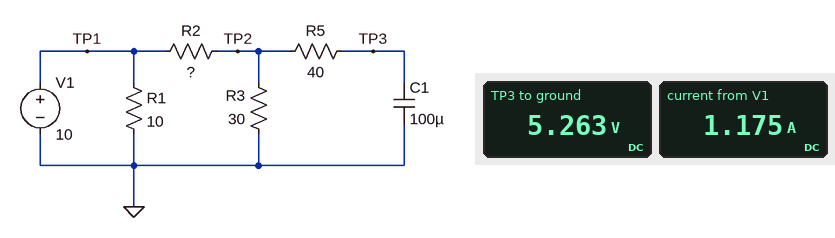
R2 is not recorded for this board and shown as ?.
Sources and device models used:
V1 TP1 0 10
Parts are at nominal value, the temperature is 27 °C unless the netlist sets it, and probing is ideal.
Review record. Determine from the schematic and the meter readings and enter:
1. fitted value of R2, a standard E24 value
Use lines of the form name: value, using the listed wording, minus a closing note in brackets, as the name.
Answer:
fitted value of R2, a standard E24 value: 27 Ω
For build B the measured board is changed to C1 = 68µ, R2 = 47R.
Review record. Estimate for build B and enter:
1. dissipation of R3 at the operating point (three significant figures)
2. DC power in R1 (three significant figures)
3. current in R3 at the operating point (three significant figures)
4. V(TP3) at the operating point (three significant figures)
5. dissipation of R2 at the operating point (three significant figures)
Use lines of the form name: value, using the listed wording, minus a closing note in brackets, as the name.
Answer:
dissipation of R3 at the operating point: 506 mW
DC power in R1: 10.0 W
current in R3 at the operating point: 130 mA
V(TP3) at the operating point: 3.90 V
dissipation of R2 at the operating point: 793 mW
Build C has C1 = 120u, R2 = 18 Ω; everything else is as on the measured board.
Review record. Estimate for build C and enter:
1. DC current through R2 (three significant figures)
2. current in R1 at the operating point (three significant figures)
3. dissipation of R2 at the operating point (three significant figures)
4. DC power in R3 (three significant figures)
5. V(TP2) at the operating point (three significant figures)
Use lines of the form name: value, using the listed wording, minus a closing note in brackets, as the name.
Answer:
DC current through R2: 208 mA
current in R1 at the operating point: 1.00 A
dissipation of R2 at the operating point: 781 mW
DC power in R3: 1.30 W
V(TP2) at the operating point: 6.25 V
